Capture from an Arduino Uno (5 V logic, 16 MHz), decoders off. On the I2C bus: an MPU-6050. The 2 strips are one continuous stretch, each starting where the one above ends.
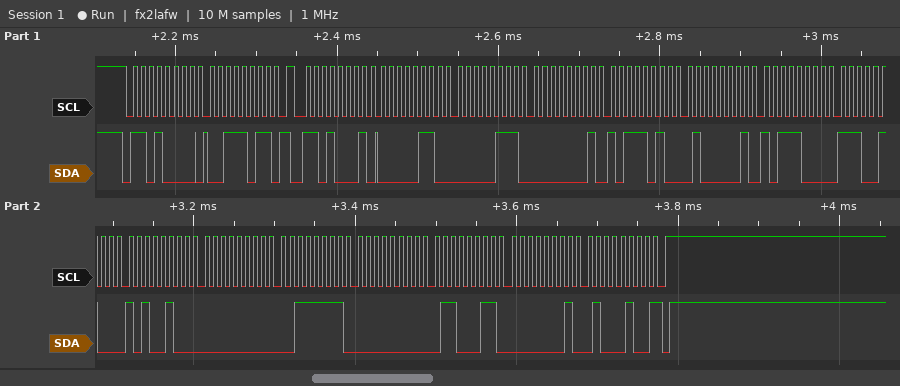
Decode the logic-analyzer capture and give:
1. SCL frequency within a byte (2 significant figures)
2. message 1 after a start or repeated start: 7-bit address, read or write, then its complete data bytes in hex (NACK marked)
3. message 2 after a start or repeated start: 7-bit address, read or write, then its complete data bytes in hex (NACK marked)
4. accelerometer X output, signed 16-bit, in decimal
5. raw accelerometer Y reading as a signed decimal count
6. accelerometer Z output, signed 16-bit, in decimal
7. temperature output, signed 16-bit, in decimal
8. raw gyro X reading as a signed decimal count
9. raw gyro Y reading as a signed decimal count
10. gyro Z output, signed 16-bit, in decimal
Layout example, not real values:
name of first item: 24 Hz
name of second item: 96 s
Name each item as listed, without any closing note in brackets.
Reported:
SCL frequency within a byte: 100 kHz
message 1 after a start or repeated start: 7-bit address, read or write, then its complete data bytes in hex: 0x68 write: 3B
message 2 after a start or repeated start: 7-bit address, read or write, then its complete data bytes in hex: 0x68 read: 06 07 01 BA 41 B8 E4 A4 00 3F 00 63 01 44 NACK
accelerometer X output, signed 16-bit, in decimal: 1543
raw accelerometer Y reading as a signed decimal count: 442
accelerometer Z output, signed 16-bit, in decimal: 16824
temperature output, signed 16-bit, in decimal: -7004
raw gyro X reading as a signed decimal count: 63
raw gyro Y reading as a signed decimal count: 99
gyro Z output, signed 16-bit, in decimal: 324
